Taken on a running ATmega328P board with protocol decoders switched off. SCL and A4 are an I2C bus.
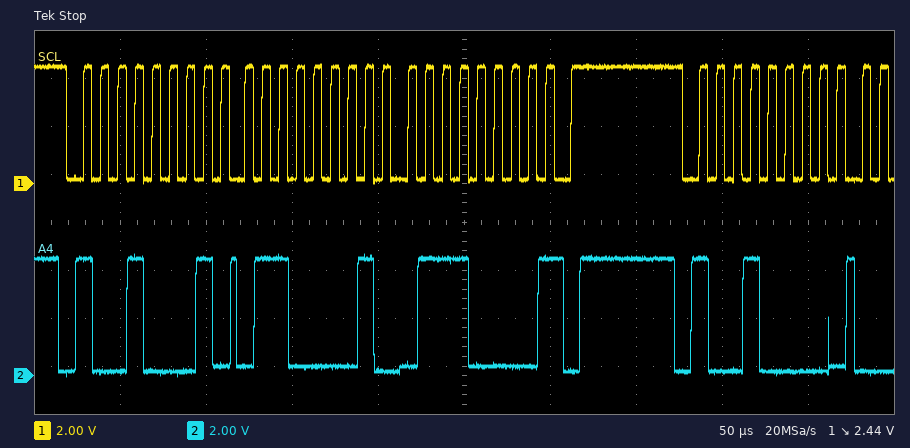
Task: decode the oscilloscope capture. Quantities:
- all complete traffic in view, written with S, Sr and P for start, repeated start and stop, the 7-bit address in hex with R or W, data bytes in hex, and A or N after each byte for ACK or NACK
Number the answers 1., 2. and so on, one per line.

1. S 48R A 61 A 70 N P S 48W A
